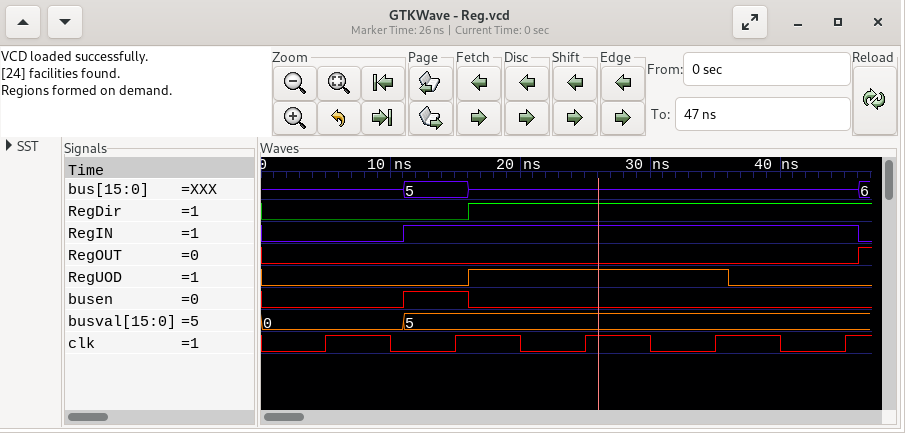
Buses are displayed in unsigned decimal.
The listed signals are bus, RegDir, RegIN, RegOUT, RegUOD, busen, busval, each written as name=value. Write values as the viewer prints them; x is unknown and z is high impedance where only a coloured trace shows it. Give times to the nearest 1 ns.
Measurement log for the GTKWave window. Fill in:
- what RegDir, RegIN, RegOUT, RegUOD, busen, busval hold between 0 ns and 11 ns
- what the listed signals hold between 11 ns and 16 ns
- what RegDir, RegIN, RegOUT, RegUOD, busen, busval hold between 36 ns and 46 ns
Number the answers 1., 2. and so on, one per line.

1. RegDir=0, RegIN=0, RegOUT=0, RegUOD=0, busen=0, busval=0
2. bus=5, RegDir=0, RegIN=1, RegOUT=0, RegUOD=0, busen=1, busval=5
3. RegDir=1, RegIN=1, RegOUT=0, RegUOD=0, busen=0, busval=5
